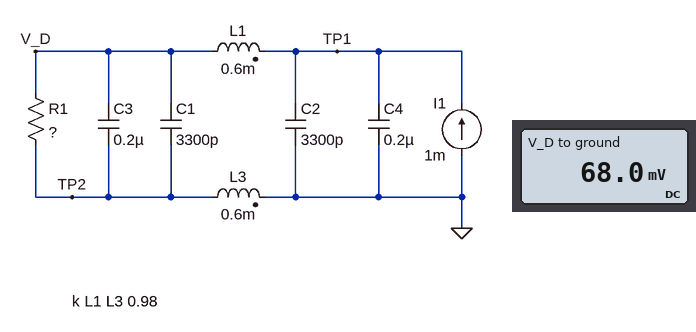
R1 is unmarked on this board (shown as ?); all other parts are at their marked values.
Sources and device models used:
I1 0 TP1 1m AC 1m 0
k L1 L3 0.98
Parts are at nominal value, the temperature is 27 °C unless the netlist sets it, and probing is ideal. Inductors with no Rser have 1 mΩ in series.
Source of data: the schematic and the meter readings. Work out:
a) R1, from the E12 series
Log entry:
68 Ω
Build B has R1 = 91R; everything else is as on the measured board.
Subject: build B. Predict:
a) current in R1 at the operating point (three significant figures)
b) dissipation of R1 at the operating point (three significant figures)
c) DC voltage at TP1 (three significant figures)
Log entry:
1.00 mA
91.0 µW
91.0 mV
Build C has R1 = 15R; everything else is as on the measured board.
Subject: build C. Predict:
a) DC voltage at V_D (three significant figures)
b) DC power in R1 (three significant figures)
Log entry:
15.0 mV
15.0 µW
